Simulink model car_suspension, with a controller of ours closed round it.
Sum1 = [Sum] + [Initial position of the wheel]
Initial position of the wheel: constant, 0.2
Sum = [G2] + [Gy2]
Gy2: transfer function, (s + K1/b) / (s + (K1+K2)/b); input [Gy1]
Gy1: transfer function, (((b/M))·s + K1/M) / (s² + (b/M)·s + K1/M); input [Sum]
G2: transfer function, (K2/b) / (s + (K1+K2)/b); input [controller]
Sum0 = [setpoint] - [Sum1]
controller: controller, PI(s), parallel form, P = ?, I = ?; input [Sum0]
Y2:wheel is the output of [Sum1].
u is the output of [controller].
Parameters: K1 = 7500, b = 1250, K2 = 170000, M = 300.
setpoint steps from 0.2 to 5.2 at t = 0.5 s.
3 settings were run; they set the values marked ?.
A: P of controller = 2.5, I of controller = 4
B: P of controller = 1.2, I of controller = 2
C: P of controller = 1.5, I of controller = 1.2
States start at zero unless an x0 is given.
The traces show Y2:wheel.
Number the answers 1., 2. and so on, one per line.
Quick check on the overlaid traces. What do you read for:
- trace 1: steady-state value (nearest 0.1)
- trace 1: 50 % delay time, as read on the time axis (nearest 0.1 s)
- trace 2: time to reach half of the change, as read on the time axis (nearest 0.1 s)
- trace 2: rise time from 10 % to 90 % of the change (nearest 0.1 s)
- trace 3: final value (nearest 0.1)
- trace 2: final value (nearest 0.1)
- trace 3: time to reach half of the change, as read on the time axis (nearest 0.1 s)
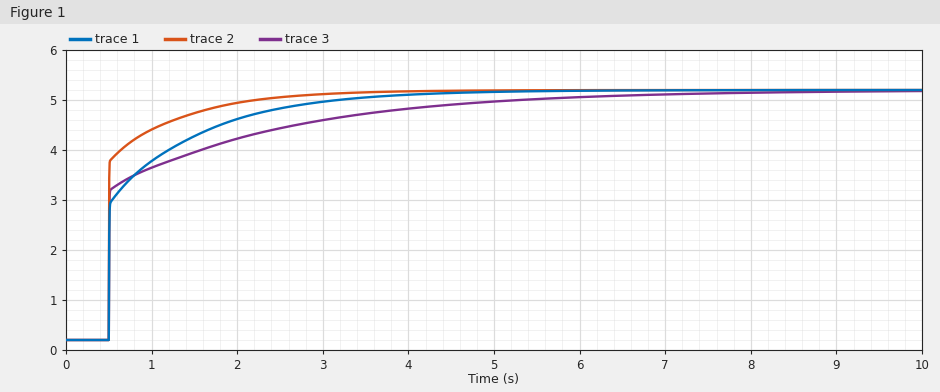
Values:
1. 5.2
2. 0.5 s
3. 0.5 s
4. 0.9 s
5. 5.2
6. 5.2
7. 0.5 s
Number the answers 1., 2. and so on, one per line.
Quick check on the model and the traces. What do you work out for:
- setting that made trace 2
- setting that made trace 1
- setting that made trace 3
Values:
1. A
2. B
3. C
